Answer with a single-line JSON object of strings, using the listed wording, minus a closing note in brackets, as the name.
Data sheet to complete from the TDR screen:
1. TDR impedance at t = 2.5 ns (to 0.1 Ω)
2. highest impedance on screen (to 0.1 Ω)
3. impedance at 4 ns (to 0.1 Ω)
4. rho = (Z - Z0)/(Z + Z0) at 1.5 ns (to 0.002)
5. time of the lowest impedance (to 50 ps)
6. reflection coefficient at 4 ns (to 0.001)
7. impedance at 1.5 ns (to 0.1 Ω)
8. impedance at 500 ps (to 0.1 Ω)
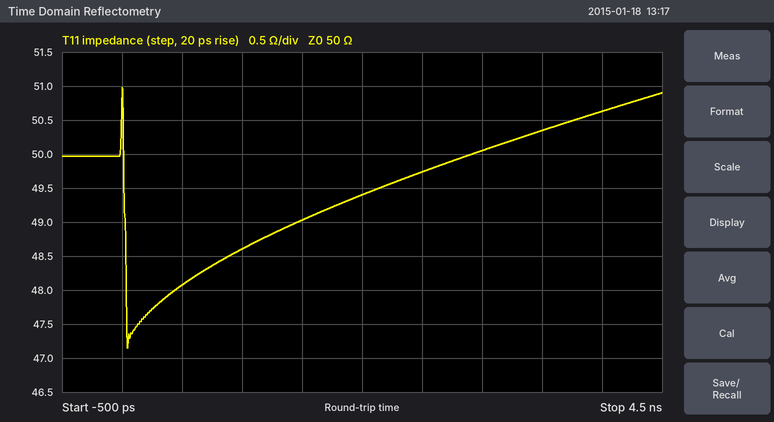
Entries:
{"TDR impedance at t = 2.5 ns": "49.7 Ω", "highest impedance on screen": "51.0 Ω", "impedance at 4 ns": "50.6 Ω", "rho = (Z - Z0)/(Z + Z0) at 1.5 ns": "-0.010", "time of the lowest impedance": "50 ps", "reflection coefficient at 4 ns": "+0.006", "impedance at 1.5 ns": "49.0 Ω", "impedance at 500 ps": "48.1 Ω"}
